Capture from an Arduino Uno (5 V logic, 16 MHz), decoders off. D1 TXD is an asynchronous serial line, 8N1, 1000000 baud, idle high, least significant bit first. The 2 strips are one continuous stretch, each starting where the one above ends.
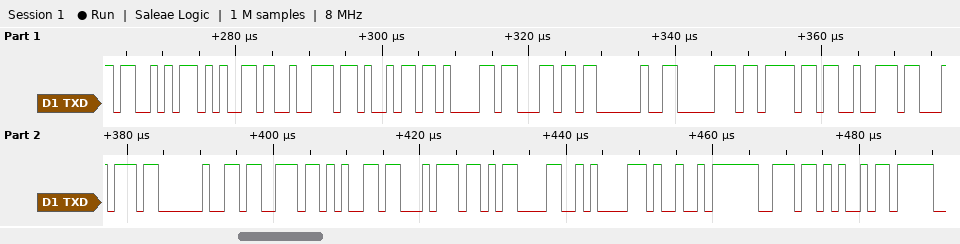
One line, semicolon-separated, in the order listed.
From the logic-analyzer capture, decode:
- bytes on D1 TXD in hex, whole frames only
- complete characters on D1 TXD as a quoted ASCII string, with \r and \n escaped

53 65 72 69 61 6C 20 70 6F 72 74 20 73 65 74 0D 0A 49 6E 69; "Serial port set\r\nIni"
